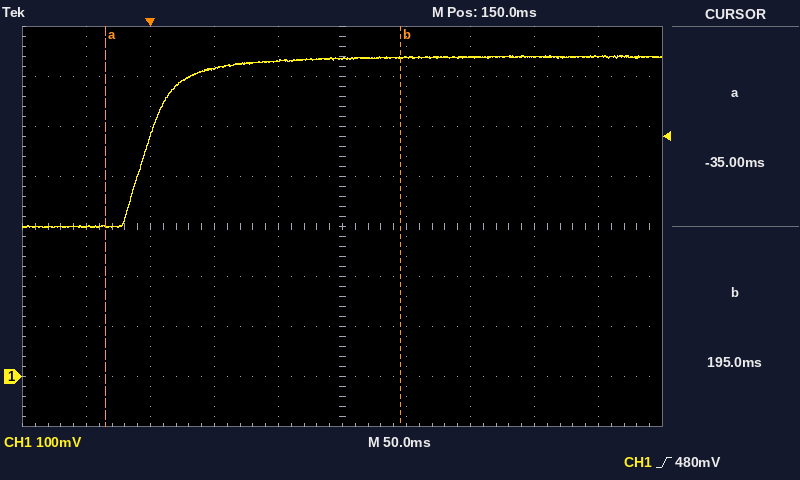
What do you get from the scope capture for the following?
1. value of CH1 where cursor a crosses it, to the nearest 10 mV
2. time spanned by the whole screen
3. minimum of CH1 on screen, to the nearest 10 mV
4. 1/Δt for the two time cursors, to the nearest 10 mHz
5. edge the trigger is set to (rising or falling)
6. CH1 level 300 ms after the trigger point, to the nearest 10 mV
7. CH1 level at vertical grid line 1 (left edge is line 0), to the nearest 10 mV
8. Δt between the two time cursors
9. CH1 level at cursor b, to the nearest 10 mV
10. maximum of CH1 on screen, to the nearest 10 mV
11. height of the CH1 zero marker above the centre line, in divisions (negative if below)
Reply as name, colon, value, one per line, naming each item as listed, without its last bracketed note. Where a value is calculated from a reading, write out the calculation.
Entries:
value of CH1 where cursor a crosses it, to the nearest 10 mV: 300 mV
time spanned by the whole screen: 500 ms
minimum of CH1 on screen, to the nearest 10 mV: 300 mV
1/Δt for the two time cursors, to the nearest 10 mHz: 1 / 230 ms ≈ 4.35 Hz
edge the trigger is set to: rising
CH1 level 300 ms after the trigger point, to the nearest 10 mV: 640 mV
CH1 level at vertical grid line 1 (left edge is line 0), to the nearest 10 mV: 300 mV
Δt between the two time cursors: 195 ms − (-35 ms) = 230 ms
CH1 level at cursor b, to the nearest 10 mV: 640 mV
maximum of CH1 on screen, to the nearest 10 mV: 640 mV
height of the CH1 zero marker above the centre line, in divisions: -3.0 div
